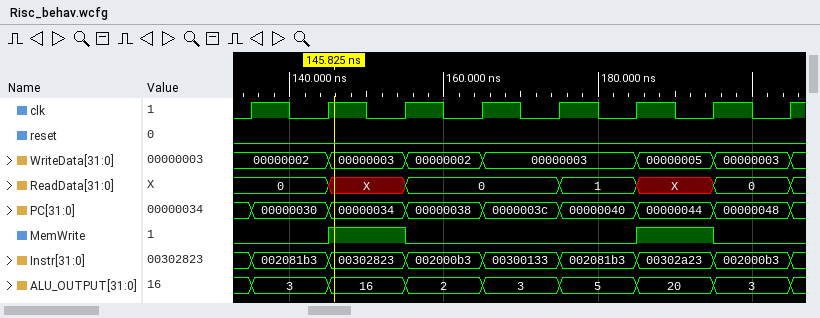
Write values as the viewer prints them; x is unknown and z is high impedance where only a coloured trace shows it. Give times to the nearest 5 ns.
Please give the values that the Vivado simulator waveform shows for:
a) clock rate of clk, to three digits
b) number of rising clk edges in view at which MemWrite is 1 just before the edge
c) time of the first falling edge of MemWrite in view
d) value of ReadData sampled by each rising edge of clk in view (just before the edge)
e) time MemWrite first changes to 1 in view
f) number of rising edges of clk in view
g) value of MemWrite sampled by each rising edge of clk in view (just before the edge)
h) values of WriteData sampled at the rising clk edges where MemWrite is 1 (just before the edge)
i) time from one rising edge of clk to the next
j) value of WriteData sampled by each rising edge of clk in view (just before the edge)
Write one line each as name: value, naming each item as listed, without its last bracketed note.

clock rate of clk, to three digits: 100 MHz
number of rising clk edges in view at which MemWrite is 1 just before the edge: 2
time of the first falling edge of MemWrite in view: 155 ns
value of ReadData sampled by each rising edge of clk in view: 0, 0, X, 0, 0, 1, X, 0
time MemWrite first changes to 1 in view: 145 ns
number of rising edges of clk in view: 8
value of MemWrite sampled by each rising edge of clk in view: 0 0 1 0 0 0 1 0
values of WriteData sampled at the rising clk edges where MemWrite is 1: 00000003, 00000005
time from one rising edge of clk to the next: 10 ns
value of WriteData sampled by each rising edge of clk in view: 00000002, 00000002, 00000003, 00000002, 00000003, 00000003, 00000005, 00000003
